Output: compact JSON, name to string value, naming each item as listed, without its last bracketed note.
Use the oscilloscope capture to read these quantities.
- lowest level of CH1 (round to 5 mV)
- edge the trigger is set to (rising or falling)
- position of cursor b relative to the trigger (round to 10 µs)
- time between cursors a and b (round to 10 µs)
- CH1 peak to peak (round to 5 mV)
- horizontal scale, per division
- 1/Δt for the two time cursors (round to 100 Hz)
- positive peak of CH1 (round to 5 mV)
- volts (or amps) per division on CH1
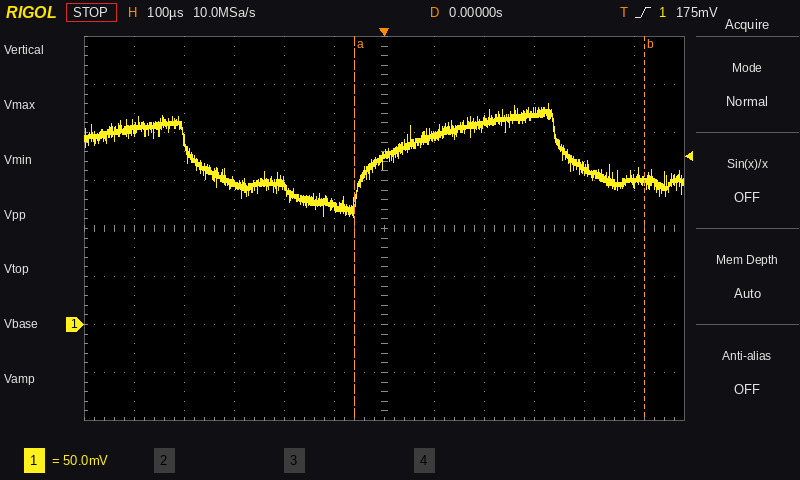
{"lowest level of CH1": "110 mV", "edge the trigger is set to": "rising", "position of cursor b relative to the trigger": "+520 µs", "time between cursors a and b": "580 µs", "CH1 peak to peak": "120 mV", "horizontal scale, per division": "100 µs", "1/Δt for the two time cursors": "1.7 kHz", "positive peak of CH1": "230 mV", "volts (or amps) per division on CH1": "50 mV"}
